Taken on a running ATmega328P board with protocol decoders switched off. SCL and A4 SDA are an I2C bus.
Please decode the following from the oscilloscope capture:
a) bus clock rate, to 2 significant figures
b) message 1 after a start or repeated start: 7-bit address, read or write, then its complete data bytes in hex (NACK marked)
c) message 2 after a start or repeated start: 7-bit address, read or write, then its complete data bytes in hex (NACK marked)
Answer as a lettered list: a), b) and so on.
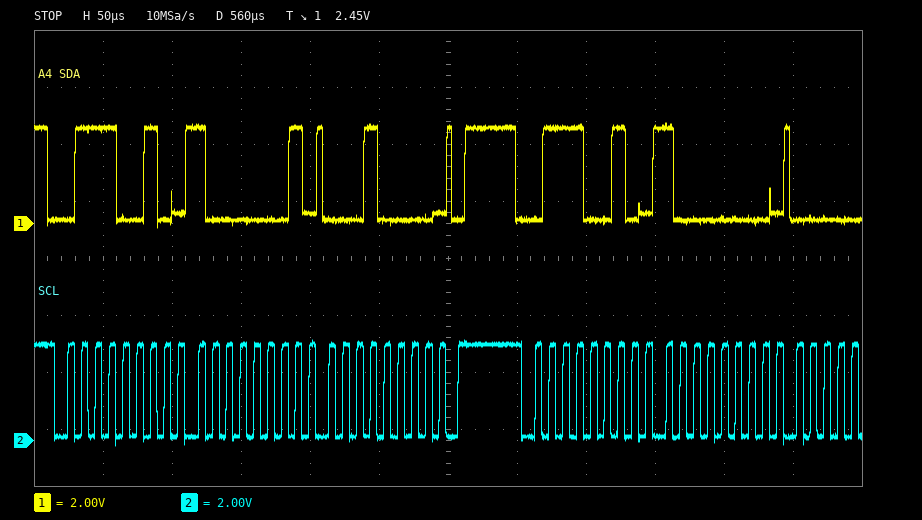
a) 100 kHz
b) 0x39 write: 81 10
c) 0x39 write: 80
